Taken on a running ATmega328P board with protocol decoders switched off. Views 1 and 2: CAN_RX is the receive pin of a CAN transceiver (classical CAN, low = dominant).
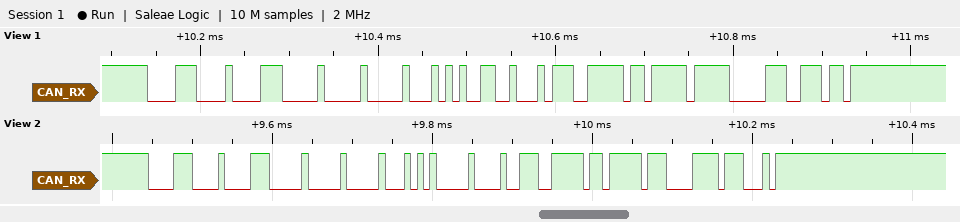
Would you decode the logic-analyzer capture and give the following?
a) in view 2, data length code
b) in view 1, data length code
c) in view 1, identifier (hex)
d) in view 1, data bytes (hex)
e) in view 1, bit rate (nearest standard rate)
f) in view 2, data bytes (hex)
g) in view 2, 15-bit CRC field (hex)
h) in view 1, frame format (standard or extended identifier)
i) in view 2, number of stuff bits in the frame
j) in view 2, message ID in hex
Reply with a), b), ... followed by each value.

a) 7
b) 7
c) 0x0E1
d) 00 00 2A 64 5C FE FF
e) 125 kbit/s
f) 00 00 2A 00 9C FE FF
g) 0x07B8
h) standard
i) 6
j) 0x0E1
